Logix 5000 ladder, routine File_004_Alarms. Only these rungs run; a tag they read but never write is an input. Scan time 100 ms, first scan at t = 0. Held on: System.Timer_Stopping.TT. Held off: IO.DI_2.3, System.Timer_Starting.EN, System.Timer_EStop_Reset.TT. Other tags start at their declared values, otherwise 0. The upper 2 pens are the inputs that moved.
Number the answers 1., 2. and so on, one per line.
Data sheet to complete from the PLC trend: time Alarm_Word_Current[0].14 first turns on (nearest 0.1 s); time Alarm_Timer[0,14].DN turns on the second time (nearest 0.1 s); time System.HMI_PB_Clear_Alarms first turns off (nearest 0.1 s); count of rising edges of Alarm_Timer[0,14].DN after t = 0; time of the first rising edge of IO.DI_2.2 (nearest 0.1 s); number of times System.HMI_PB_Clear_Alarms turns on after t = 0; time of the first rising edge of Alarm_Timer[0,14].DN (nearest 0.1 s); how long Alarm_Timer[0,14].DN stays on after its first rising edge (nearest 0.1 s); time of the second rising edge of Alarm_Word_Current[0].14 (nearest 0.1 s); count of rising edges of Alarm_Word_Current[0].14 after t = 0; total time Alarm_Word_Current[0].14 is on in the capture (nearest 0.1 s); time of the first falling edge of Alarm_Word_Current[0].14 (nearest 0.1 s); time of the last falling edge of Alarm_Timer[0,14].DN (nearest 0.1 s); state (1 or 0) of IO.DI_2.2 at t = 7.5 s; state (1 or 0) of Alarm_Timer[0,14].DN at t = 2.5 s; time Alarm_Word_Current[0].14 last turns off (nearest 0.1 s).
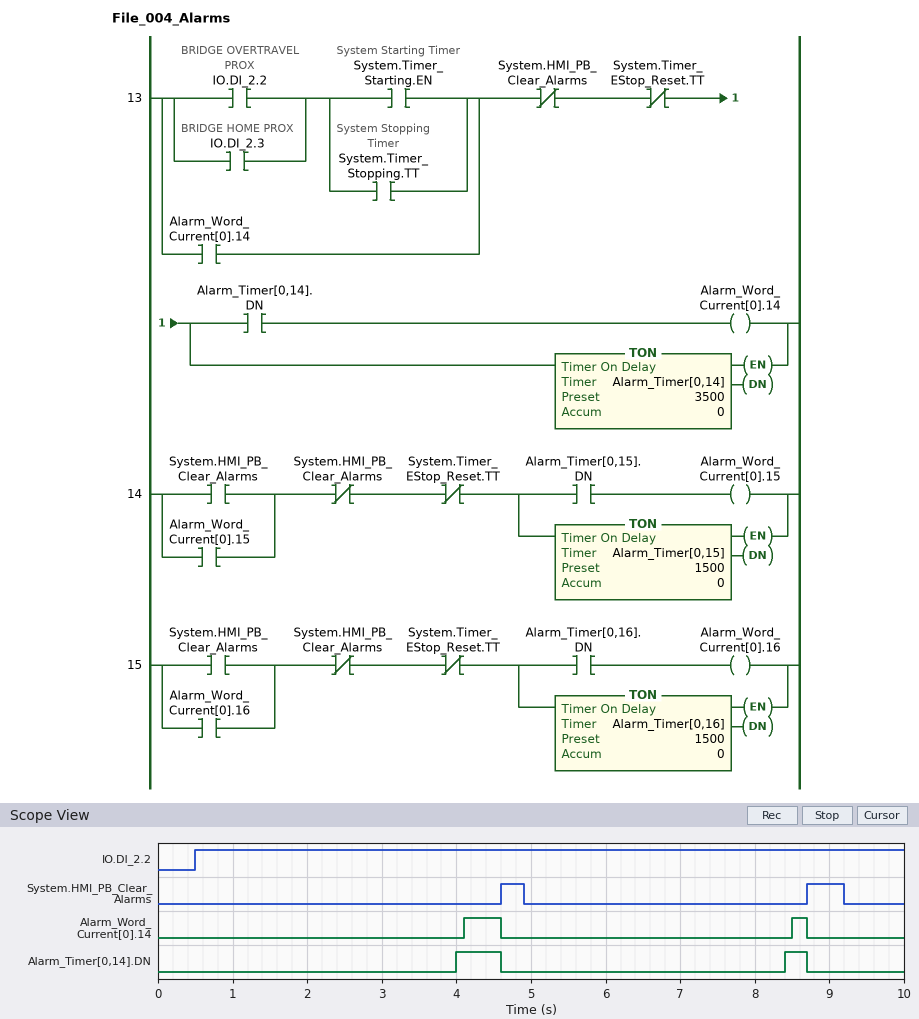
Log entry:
1. 4.1 s
2. 8.4 s
3. 4.9 s
4. 2
5. 0.5 s
6. 2
7. 4.0 s
8. 0.6 s
9. 8.5 s
10. 2
11. 0.7 s
12. 4.6 s
13. 8.7 s
14. 1
15. 0
16. 8.7 s
